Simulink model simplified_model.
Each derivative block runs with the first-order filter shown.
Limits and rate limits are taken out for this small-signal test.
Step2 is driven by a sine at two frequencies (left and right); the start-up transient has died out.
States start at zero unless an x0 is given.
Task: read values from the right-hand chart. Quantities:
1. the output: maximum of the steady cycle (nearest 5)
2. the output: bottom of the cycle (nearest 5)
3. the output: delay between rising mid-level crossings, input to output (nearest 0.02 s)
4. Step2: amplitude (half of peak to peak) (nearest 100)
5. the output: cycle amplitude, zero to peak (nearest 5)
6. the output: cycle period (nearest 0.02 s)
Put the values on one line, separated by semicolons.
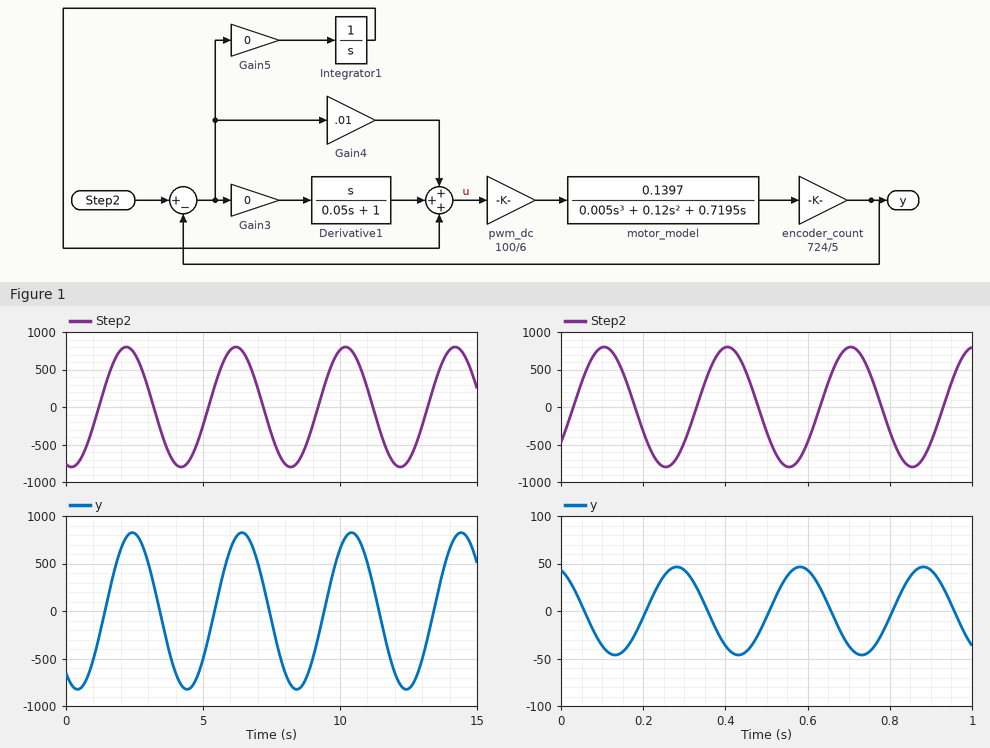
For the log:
45; -45; 0.18 s; 800; 45; 0.30 s
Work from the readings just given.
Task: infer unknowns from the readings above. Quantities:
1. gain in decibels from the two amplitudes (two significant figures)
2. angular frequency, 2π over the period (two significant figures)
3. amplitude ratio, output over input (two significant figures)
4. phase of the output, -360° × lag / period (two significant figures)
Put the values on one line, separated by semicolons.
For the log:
-25 dB; 21 rad/s; 0.056; -220°
